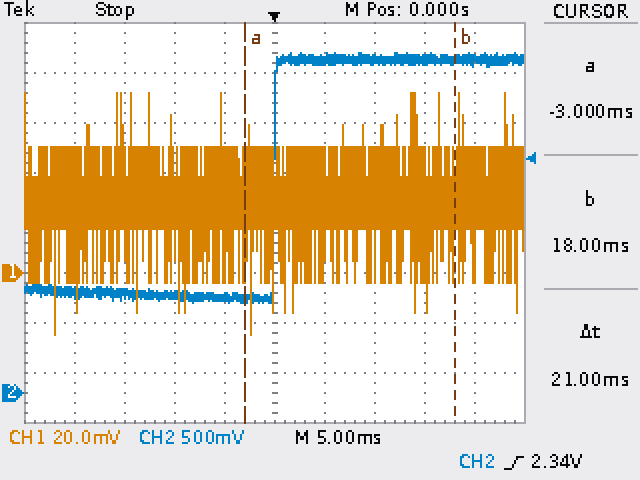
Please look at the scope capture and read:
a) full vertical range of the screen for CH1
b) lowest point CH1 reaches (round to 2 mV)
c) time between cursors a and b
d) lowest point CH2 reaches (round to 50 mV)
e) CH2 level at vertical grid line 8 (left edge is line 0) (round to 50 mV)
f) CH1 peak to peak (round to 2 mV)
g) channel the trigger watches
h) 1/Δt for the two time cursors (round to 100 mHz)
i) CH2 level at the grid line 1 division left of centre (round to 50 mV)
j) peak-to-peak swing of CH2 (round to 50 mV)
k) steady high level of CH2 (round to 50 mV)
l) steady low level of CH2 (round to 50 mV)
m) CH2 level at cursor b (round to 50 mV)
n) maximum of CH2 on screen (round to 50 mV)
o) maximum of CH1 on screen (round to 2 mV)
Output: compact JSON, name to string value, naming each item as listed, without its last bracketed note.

{"full vertical range of the screen for CH1": "160 mV", "lowest point CH1 reaches": "-24 mV", "time between cursors a and b": "21 ms", "lowest point CH2 reaches": "900 mV", "CH2 level at vertical grid line 8 (left edge is line 0)": "3.35 V", "CH1 peak to peak": "96 mV", "channel the trigger watches": "CH2", "1/Δt for the two time cursors": "47.6 Hz", "CH2 level at the grid line 1 division left of centre": "950 mV", "peak-to-peak swing of CH2": "2.50 V", "steady high level of CH2": "3.35 V", "steady low level of CH2": "1.00 V", "CH2 level at cursor b": "3.35 V", "maximum of CH2 on screen": "3.40 V", "maximum of CH1 on screen": "72 mV"}
